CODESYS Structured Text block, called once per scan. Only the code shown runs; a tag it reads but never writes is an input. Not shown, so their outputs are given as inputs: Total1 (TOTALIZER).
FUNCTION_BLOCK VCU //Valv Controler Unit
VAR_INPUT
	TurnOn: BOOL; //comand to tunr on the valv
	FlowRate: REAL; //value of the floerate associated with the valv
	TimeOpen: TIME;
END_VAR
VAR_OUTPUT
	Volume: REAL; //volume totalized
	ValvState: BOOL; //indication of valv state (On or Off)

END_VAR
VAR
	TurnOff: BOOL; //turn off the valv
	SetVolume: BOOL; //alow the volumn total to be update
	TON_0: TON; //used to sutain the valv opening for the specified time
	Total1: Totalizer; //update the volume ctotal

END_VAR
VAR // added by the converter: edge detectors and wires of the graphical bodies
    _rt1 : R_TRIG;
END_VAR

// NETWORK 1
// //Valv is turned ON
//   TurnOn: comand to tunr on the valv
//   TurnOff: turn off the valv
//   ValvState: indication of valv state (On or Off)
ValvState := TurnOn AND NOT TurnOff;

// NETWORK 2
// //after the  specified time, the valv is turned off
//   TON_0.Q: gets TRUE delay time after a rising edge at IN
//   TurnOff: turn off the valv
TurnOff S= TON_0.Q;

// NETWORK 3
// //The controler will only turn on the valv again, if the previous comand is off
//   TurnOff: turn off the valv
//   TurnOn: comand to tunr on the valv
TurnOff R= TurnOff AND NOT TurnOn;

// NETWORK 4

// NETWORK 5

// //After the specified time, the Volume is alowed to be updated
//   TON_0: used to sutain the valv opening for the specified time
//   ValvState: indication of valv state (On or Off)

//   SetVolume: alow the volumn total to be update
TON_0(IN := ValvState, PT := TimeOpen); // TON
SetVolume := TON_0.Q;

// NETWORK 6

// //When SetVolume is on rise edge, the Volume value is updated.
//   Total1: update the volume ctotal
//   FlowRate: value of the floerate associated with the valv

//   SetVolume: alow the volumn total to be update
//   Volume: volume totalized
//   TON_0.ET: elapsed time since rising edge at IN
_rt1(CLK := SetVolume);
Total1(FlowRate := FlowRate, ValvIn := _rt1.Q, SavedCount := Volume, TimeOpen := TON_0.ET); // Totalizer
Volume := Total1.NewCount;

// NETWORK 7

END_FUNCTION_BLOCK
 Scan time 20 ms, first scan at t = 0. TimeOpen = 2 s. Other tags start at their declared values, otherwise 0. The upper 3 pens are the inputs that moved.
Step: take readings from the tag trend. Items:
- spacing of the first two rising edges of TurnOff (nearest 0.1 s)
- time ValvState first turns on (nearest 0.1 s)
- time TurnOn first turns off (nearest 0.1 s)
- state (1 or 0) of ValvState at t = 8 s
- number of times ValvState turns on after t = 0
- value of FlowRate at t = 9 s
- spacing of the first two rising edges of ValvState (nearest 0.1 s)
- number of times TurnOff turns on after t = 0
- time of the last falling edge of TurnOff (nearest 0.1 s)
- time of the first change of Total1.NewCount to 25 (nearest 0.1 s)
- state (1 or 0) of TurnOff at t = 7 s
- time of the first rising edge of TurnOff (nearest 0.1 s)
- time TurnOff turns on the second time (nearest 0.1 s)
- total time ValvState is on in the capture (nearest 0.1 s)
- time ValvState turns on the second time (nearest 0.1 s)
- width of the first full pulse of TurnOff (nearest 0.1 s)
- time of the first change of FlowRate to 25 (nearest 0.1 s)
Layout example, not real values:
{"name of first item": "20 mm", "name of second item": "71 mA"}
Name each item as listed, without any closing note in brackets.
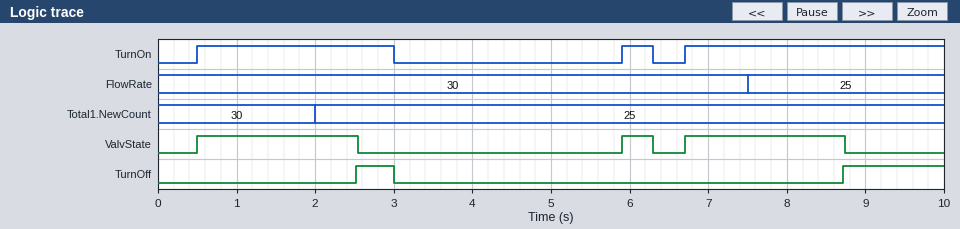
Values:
{"spacing of the first two rising edges of TurnOff": "6.2 s", "time ValvState first turns on": "0.5 s", "time TurnOn first turns off": "3.0 s", "state (1 or 0) of ValvState at t = 8 s": "1", "number of times ValvState turns on after t = 0": "3", "value of FlowRate at t = 9 s": "25", "spacing of the first two rising edges of ValvState": "5.4 s", "number of times TurnOff turns on after t = 0": "2", "time of the last falling edge of TurnOff": "3.0 s", "time of the first change of Total1.NewCount to 25": "2.0 s", "state (1 or 0) of TurnOff at t = 7 s": "0", "time of the first rising edge of TurnOff": "2.5 s", "time TurnOff turns on the second time": "8.7 s", "total time ValvState is on in the capture": "4.5 s", "time ValvState turns on the second time": "5.9 s", "width of the first full pulse of TurnOff": "0.5 s", "time of the first change of FlowRate to 25": "7.5 s"}
